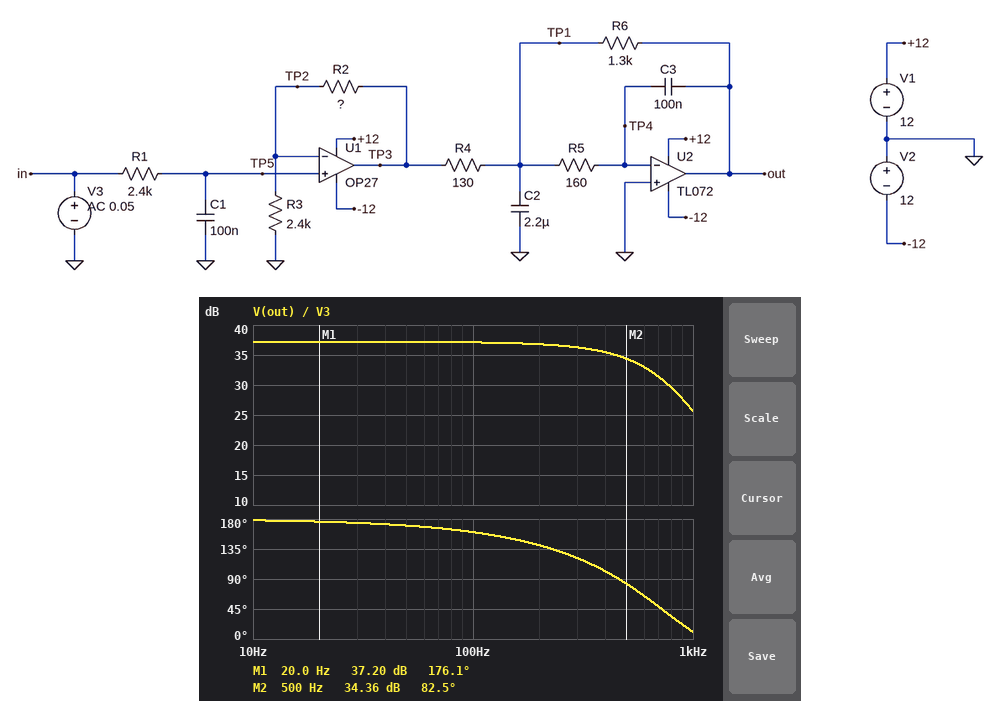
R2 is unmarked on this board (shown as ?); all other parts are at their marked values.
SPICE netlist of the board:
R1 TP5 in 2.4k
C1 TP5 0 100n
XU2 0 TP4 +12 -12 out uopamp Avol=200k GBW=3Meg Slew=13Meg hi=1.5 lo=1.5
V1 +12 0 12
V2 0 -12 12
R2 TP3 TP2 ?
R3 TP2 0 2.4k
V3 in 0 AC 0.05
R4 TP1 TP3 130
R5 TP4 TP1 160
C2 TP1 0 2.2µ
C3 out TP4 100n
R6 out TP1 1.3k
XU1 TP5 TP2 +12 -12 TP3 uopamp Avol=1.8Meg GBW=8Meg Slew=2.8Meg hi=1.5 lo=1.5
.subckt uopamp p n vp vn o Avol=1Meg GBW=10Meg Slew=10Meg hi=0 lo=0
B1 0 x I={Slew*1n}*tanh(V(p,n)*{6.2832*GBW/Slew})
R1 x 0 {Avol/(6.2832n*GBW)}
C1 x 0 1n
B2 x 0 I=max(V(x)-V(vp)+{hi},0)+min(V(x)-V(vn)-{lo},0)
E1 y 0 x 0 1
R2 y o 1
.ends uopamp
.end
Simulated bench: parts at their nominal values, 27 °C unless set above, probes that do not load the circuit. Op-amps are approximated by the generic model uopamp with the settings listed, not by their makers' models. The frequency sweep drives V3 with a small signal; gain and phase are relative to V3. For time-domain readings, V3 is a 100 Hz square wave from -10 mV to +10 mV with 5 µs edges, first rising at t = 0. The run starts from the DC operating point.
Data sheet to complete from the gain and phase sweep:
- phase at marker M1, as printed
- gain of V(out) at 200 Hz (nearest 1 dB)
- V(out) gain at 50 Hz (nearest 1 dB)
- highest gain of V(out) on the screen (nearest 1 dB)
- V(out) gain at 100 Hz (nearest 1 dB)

176.1 deg
37 dB
37 dB
37 dB
37 dB
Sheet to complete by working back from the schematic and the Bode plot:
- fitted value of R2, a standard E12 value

15 kΩ
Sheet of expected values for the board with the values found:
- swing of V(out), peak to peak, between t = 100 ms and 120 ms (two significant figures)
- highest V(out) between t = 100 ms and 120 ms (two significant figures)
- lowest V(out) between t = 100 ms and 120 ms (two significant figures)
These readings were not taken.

1.5 V
740 mV
-740 mV
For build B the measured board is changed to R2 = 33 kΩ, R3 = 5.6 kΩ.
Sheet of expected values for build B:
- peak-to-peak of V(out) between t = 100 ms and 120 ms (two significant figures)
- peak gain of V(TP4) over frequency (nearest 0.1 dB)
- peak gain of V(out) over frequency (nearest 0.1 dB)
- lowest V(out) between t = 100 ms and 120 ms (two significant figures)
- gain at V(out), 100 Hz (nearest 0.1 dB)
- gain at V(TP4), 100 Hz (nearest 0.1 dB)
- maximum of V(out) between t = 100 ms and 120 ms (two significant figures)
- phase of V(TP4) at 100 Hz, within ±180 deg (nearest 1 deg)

1.4 V
-41.4 dB
36.8 dB
-700 mV
36.7 dB
-52.8 dB
700 mV
62 deg
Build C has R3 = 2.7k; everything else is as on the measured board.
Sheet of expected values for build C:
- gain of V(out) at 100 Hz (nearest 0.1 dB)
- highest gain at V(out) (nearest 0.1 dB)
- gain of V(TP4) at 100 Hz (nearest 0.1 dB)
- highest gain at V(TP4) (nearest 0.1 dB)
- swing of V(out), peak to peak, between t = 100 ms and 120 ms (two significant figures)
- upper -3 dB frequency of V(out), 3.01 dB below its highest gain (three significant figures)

36.2 dB
36.3 dB
-53.2 dB
-41.9 dB
1.3 V
513 Hz
